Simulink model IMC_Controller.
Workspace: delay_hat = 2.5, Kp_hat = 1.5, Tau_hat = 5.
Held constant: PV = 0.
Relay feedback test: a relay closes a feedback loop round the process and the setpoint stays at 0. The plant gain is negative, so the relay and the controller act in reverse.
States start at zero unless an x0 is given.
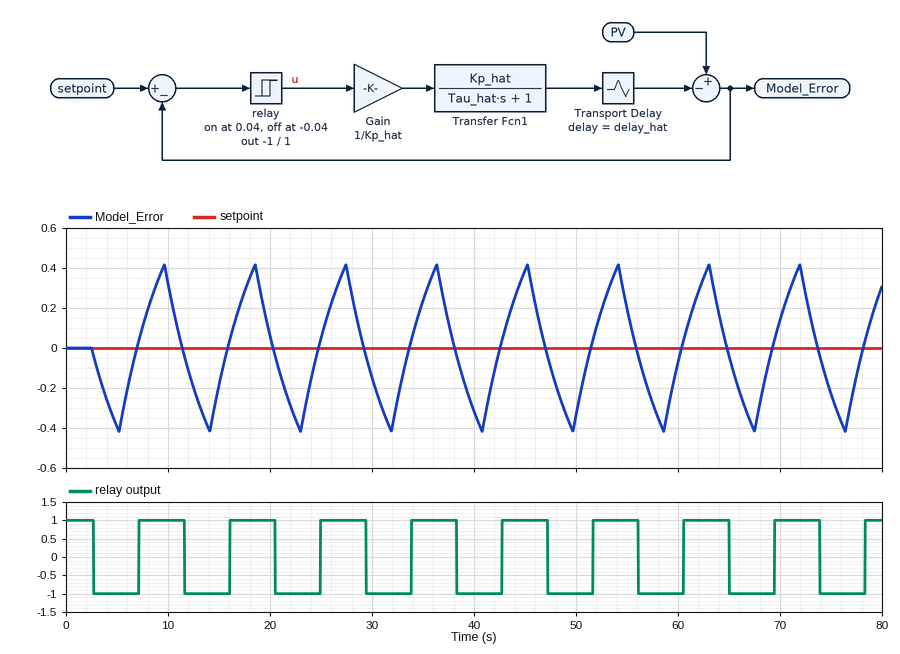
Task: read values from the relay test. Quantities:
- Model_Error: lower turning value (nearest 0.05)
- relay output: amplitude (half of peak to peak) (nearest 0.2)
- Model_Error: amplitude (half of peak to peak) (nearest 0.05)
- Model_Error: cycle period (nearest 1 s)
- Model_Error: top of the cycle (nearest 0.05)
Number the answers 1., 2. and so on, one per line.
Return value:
1. -0.40
2. 1.0
3. 0.40
4. 9 s
5. 0.40
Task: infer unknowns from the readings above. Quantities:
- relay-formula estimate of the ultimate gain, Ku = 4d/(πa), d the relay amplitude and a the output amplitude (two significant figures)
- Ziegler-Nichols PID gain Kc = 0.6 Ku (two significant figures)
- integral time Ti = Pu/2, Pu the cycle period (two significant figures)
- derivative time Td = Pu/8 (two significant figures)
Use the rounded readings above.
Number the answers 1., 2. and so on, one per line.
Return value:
1. 3.2
2. 1.9
3. 4.5 s
4. 1.1 s
